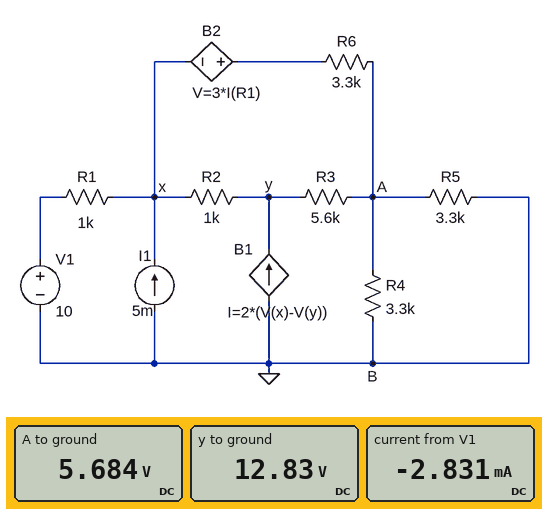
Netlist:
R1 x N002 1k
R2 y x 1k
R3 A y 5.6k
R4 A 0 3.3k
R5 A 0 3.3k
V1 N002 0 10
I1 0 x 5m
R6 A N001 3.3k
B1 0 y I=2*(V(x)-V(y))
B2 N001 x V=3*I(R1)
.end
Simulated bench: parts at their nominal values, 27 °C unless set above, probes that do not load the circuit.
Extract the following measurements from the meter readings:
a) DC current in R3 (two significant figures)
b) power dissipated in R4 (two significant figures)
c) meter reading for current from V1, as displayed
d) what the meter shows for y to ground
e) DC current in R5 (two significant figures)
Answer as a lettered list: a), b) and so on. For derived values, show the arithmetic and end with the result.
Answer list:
a) (12.83 V - 5.684 V) / 5.6 kΩ = 1.3 mA
b) (5.684 V)^2 / 3.3 kΩ = 9.8 mW
c) -2.831 mA
d) 12.83 V
e) (5.684 V) / 3.3 kΩ = 1.7 mA
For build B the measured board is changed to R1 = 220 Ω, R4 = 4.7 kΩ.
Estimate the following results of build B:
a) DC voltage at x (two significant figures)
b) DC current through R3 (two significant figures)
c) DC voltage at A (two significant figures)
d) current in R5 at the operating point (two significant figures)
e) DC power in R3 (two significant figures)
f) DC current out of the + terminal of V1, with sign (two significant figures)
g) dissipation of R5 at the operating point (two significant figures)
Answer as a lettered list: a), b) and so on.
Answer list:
a) 11 V
b) 990 µA
c) 5.2 V
d) 1.6 mA
e) 5.5 mW
f) -3.3 mA
g) 8.1 mW
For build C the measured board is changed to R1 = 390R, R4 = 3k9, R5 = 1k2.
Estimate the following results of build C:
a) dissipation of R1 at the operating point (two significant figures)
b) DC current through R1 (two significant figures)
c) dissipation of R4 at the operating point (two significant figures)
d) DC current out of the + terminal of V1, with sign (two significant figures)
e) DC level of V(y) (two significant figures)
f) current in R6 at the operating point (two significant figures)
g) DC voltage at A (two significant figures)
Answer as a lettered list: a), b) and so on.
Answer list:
a) 2.8 mW
b) 2.7 mA
c) 2.9 mW
d) -2.7 mA
e) 11 V
f) 2.3 mA
g) 3.4 V
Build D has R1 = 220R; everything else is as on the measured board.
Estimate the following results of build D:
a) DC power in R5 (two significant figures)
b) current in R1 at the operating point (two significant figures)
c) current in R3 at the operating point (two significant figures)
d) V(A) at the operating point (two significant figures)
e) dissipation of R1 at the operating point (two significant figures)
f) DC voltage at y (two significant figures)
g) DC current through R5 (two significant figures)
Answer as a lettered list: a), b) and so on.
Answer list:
a) 6.8 mW
b) 3.2 mA
c) 1.1 mA
d) 4.7 V
e) 2.2 mW
f) 11 V
g) 1.4 mA
